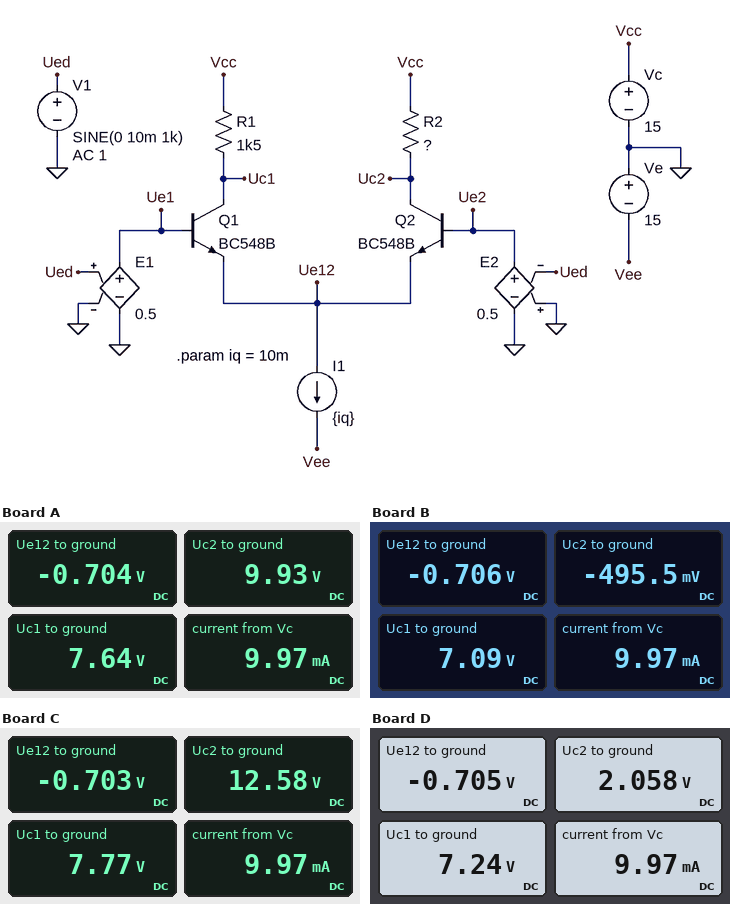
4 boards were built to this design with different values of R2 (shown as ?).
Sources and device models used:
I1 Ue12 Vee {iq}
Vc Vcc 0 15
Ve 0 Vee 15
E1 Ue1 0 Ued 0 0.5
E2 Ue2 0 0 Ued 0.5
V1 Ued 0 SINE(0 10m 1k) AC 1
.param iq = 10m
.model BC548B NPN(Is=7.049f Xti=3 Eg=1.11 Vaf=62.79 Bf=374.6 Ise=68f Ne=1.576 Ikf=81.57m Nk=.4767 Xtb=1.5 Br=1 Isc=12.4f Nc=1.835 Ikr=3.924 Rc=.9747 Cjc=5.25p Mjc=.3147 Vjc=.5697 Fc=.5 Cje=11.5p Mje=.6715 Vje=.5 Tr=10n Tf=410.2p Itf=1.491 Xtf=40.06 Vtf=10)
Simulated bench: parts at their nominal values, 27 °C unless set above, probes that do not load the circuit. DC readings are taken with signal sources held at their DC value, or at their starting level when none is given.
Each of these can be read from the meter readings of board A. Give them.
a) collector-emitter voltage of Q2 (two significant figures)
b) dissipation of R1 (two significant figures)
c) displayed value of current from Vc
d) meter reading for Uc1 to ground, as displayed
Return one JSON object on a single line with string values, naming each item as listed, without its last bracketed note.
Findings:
{"collector-emitter voltage of Q2": "11 V", "dissipation of R1": "36 mW", "displayed value of current from Vc": "9.97 mA", "meter reading for Uc1 to ground, as displayed": "7.64 V"}
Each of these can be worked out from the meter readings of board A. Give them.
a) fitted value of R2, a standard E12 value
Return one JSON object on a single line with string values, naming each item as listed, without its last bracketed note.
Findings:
{"fitted value of R2, a standard E12 value": "1 kΩ"}
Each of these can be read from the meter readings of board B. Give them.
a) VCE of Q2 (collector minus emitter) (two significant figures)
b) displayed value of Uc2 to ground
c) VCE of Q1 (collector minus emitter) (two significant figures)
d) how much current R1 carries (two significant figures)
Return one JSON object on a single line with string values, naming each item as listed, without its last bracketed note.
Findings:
{"VCE of Q2 (collector minus emitter)": "210 mV", "displayed value of Uc2 to ground": "-495.5 mV", "VCE of Q1 (collector minus emitter)": "7.8 V", "how much current R1 carries": "5.3 mA"}
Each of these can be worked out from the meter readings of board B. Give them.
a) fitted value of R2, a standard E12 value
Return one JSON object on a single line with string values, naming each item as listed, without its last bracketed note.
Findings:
{"fitted value of R2, a standard E12 value": "3.3 kΩ"}
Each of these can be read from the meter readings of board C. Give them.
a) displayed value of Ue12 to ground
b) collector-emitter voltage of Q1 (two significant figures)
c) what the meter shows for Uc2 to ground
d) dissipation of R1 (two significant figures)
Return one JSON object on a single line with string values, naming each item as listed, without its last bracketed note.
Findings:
{"displayed value of Ue12 to ground": "-0.703 V", "collector-emitter voltage of Q1": "8.5 V", "what the meter shows for Uc2 to ground": "12.58 V", "dissipation of R1": "35 mW"}
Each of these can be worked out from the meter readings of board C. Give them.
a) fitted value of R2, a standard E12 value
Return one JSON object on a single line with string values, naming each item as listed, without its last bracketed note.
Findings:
{"fitted value of R2, a standard E12 value": "470 Ω"}
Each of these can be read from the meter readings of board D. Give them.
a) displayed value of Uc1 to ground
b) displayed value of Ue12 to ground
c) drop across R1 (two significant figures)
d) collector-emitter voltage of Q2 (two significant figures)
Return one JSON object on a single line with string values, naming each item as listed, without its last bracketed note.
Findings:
{"displayed value of Uc1 to ground": "7.24 V", "displayed value of Ue12 to ground": "-0.705 V", "drop across R1": "7.8 V", "collector-emitter voltage of Q2": "2.8 V"}
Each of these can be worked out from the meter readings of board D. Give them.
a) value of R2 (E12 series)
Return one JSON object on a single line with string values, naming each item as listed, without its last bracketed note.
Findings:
{"value of R2": "2.7 kΩ"}
